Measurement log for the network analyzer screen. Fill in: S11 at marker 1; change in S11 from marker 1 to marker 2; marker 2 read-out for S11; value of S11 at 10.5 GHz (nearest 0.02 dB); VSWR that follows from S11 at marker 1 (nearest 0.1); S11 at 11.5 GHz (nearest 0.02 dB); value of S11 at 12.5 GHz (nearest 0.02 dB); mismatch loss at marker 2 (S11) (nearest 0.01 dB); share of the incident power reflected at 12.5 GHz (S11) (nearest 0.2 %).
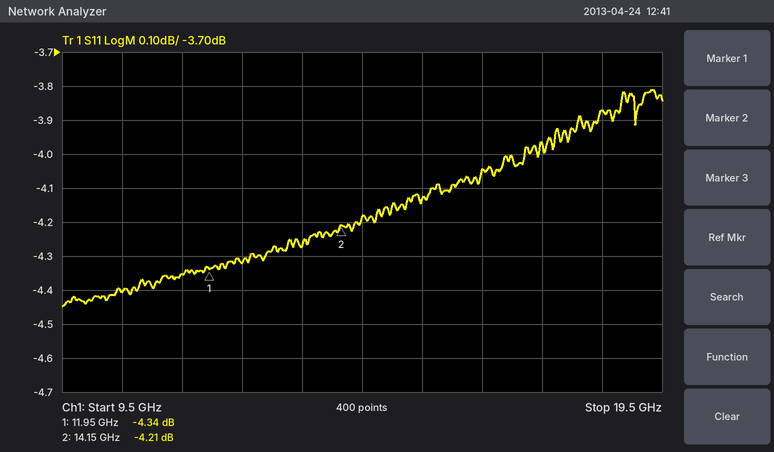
-4.34 dB
0.13 dB
-4.21 dB
-4.40 dB
4.1
-4.36 dB
-4.32 dB
2.07 dB
37.0 %
